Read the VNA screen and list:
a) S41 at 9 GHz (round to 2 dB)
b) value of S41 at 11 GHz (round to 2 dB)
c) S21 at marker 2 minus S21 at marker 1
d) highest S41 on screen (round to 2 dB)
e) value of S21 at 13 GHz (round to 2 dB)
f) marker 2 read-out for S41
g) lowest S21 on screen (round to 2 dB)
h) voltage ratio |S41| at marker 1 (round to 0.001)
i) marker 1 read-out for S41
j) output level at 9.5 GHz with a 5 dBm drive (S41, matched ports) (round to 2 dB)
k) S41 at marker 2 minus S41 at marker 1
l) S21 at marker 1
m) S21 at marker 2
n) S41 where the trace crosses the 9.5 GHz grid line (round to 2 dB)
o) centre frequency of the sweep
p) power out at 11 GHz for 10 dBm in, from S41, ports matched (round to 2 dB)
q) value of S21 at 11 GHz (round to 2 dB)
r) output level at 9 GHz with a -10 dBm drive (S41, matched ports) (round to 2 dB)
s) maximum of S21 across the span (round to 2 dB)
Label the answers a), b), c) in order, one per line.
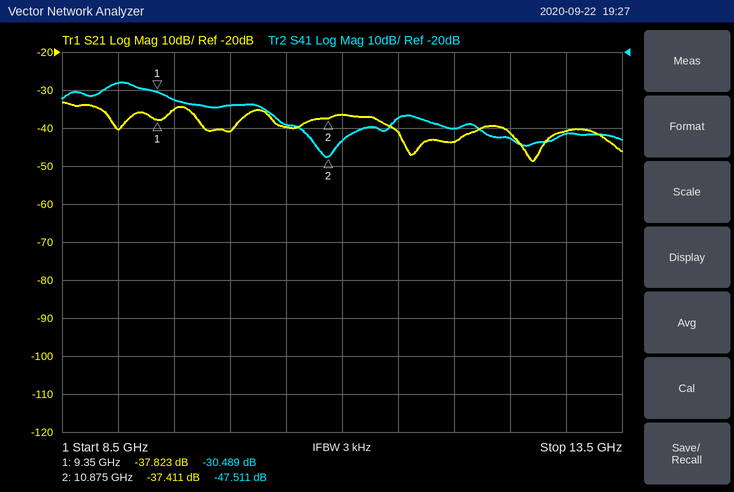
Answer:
a) -28 dB
b) -44 dB
c) 0.412 dB
d) -28 dB
e) -40 dB
f) -47.511 dB
g) -48 dB
h) 0.030
i) -30.489 dB
j) -28 dBm
k) -17.022 dB
l) -37.823 dB
m) -37.411 dB
n) -32 dB
o) 11 GHz
p) -34 dBm
q) -36 dB
r) -38 dBm
s) -34 dB
